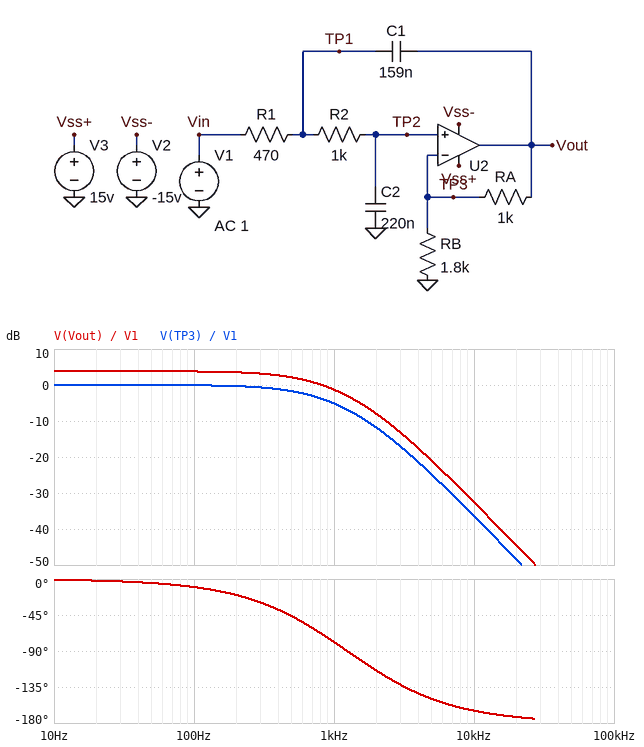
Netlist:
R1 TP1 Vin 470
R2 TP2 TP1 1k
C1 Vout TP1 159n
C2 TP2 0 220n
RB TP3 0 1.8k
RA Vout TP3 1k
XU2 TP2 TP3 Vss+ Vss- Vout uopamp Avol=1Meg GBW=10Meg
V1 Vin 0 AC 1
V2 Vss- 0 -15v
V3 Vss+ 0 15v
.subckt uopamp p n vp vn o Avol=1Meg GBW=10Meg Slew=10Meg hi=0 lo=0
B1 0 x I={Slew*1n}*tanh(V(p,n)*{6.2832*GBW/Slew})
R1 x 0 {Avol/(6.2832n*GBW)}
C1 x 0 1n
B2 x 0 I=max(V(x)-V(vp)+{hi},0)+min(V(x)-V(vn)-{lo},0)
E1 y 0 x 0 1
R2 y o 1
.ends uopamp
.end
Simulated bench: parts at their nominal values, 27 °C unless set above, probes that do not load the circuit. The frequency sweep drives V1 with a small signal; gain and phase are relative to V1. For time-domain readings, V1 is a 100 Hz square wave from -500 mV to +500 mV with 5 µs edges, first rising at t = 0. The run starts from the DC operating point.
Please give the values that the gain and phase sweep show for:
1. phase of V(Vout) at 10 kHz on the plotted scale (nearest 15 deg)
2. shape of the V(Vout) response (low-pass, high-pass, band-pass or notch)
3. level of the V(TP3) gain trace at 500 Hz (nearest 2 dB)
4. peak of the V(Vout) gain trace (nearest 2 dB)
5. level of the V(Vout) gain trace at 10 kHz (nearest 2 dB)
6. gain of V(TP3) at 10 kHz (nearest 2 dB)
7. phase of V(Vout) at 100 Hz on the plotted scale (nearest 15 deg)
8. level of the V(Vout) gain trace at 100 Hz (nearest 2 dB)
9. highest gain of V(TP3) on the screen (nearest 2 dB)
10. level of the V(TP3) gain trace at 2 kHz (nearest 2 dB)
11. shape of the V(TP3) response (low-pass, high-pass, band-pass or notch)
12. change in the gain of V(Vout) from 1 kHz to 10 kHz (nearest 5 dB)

-165 deg
low-pass
-2 dB
4 dB
-32 dB
-36 dB
-15 deg
4 dB
0 dB
-12 dB
low-pass
-30 dB
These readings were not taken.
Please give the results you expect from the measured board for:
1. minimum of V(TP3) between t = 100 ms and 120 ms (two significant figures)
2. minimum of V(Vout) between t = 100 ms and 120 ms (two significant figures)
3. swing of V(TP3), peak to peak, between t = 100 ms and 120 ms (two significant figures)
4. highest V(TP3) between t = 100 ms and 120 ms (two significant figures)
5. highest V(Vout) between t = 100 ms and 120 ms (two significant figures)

-500 mV
-780 mV
1.0 V
500 mV
780 mV
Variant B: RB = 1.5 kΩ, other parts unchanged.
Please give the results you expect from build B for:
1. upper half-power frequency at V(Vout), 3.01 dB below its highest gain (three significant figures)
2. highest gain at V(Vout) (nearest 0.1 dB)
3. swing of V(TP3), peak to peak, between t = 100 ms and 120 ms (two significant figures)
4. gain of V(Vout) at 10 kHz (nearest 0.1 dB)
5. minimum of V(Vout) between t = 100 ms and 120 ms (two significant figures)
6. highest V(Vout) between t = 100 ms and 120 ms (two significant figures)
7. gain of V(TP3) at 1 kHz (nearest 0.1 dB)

729 Hz
4.4 dB
1.0 V
-32.0 dB
-830 mV
830 mV
-4.9 dB
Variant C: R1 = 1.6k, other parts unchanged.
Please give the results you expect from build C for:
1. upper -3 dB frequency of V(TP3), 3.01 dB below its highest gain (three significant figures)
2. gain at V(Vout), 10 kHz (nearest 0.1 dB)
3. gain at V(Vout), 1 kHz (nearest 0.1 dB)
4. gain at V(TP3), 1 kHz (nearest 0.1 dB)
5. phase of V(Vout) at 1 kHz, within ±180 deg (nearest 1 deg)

494 Hz
-43.1 dB
-5.6 dB
-9.4 dB
-114 deg
